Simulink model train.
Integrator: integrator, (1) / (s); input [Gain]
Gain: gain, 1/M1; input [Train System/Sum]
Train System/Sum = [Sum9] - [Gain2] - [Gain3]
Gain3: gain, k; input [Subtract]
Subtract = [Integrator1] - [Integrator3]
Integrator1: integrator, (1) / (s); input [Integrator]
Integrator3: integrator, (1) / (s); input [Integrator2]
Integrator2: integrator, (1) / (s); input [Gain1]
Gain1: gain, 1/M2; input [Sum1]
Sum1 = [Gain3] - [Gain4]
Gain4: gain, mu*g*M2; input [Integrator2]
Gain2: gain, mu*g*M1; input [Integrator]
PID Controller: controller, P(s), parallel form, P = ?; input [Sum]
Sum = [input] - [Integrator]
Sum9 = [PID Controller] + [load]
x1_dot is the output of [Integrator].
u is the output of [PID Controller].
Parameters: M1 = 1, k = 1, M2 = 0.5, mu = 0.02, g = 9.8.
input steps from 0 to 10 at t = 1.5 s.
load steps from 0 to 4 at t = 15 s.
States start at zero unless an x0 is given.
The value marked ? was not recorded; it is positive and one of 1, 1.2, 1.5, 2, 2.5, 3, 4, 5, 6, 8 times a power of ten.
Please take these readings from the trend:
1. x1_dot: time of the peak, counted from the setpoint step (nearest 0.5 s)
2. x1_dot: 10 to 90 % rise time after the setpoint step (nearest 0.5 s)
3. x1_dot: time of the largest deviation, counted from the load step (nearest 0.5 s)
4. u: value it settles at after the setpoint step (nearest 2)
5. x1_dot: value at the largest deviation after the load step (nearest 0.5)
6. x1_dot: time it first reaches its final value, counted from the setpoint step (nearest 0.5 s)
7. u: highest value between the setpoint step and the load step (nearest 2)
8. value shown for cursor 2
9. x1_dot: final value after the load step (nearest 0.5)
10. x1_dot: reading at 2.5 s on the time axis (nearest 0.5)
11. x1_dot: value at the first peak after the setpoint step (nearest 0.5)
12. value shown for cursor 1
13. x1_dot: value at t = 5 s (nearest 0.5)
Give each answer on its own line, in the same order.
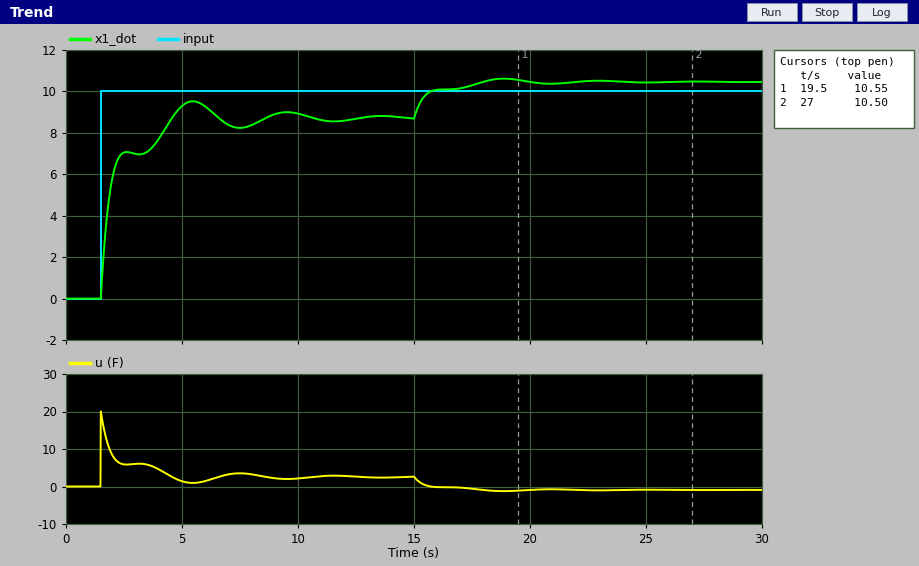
4.0 s
2.5 s
4.0 s
2
10.5
3.0 s
20
10.50
10.5
7.0
9.5
10.55
9.5
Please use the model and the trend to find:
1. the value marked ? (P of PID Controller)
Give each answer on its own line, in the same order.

2
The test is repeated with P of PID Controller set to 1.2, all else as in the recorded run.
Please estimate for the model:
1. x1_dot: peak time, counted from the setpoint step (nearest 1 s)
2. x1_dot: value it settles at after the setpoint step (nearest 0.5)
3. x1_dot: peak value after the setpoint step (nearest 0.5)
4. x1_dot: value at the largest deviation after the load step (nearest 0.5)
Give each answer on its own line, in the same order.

4 s
8.0
8.5
11.0
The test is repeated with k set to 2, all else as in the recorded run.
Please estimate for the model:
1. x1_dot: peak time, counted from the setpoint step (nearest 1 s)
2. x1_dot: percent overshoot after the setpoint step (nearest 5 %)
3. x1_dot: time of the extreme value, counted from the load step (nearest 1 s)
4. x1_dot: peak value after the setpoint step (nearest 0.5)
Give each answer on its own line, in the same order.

3 s
10 %
3 s
9.5
